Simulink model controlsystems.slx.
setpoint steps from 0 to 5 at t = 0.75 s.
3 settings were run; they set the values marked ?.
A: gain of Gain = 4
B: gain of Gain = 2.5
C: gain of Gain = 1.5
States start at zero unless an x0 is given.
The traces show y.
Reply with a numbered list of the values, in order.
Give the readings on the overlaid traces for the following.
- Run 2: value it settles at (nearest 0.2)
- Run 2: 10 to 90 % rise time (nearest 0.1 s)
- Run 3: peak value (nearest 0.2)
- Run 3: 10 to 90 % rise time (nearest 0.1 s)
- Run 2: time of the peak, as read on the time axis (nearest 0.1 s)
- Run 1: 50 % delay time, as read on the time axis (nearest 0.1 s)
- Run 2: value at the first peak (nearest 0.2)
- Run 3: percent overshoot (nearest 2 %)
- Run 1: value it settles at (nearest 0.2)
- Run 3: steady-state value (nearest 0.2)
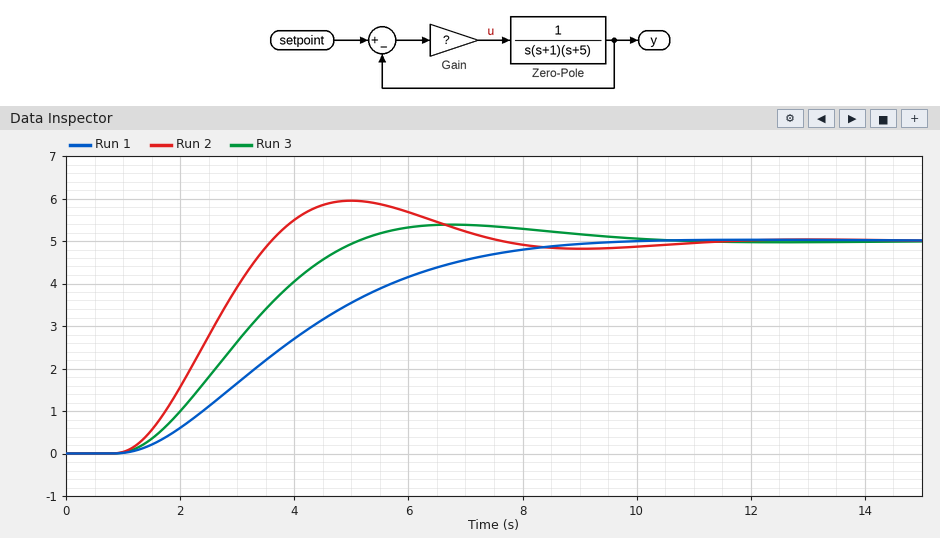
1. 5.0
2. 1.8 s
3. 5.4
4. 2.8 s
5. 5.0 s
6. 3.8 s
7. 6.0
8. 8 %
9. 5.0
10. 5.0
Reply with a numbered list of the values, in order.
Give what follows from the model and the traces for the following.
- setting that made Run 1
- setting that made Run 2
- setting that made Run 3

1. C
2. A
3. B
